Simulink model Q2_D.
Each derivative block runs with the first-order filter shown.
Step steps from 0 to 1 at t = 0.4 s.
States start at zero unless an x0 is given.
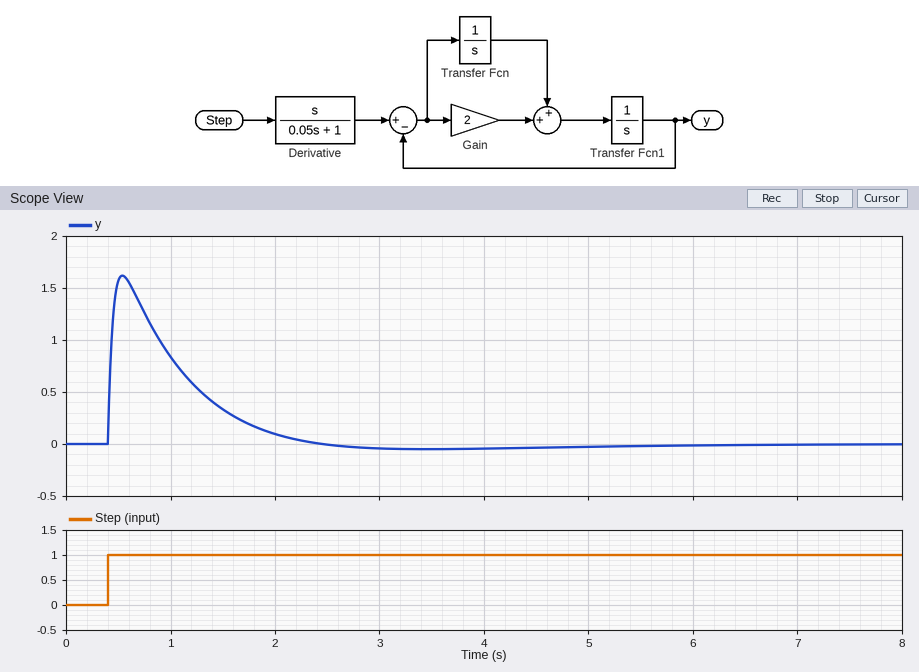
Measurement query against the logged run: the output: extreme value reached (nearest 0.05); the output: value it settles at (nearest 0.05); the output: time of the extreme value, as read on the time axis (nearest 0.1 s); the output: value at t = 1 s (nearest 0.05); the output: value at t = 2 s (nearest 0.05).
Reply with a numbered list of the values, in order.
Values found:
1. 1.60
2. 0.00
3. 0.5 s
4. 0.85
5. 0.10
